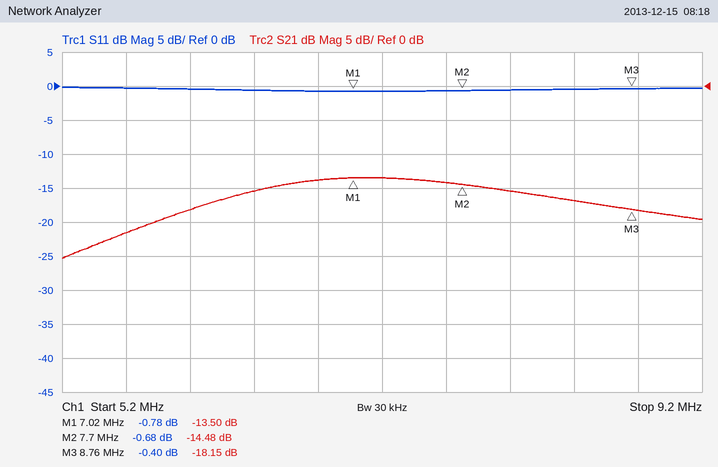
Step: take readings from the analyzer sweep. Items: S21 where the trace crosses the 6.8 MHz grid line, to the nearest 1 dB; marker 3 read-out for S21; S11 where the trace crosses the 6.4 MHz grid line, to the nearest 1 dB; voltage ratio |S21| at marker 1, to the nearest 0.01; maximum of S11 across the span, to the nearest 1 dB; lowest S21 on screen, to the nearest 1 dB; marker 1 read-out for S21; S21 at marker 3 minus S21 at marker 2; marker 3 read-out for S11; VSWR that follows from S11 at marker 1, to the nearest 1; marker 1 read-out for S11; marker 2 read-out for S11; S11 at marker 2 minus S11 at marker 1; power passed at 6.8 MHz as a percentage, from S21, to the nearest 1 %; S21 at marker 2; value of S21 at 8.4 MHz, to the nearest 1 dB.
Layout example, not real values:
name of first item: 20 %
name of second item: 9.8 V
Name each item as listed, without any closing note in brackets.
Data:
S21 where the trace crosses the 6.8 MHz grid line, to the nearest 1 dB: -14 dB
marker 3 read-out for S21: -18.15 dB
S11 where the trace crosses the 6.4 MHz grid line, to the nearest 1 dB: -1 dB
voltage ratio |S21| at marker 1, to the nearest 0.01: 0.21
maximum of S11 across the span, to the nearest 1 dB: 0 dB
lowest S21 on screen, to the nearest 1 dB: -25 dB
marker 1 read-out for S21: -13.50 dB
S21 at marker 3 minus S21 at marker 2: -3.67 dB
marker 3 read-out for S11: -0.40 dB
VSWR that follows from S11 at marker 1, to the nearest 1: 22
marker 1 read-out for S11: -0.78 dB
marker 2 read-out for S11: -0.68 dB
S11 at marker 2 minus S11 at marker 1: 0.10 dB
power passed at 6.8 MHz as a percentage, from S21, to the nearest 1 %: 4 %
S21 at marker 2: -14.48 dB
value of S21 at 8.4 MHz, to the nearest 1 dB: -17 dB
